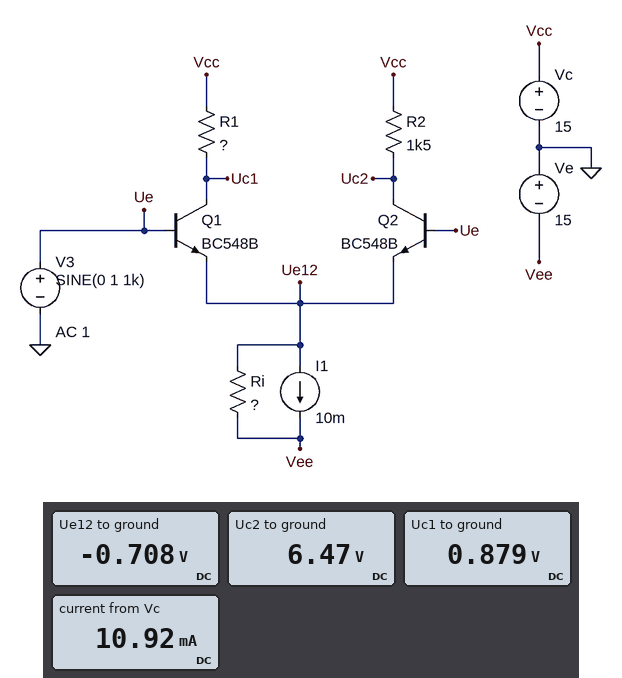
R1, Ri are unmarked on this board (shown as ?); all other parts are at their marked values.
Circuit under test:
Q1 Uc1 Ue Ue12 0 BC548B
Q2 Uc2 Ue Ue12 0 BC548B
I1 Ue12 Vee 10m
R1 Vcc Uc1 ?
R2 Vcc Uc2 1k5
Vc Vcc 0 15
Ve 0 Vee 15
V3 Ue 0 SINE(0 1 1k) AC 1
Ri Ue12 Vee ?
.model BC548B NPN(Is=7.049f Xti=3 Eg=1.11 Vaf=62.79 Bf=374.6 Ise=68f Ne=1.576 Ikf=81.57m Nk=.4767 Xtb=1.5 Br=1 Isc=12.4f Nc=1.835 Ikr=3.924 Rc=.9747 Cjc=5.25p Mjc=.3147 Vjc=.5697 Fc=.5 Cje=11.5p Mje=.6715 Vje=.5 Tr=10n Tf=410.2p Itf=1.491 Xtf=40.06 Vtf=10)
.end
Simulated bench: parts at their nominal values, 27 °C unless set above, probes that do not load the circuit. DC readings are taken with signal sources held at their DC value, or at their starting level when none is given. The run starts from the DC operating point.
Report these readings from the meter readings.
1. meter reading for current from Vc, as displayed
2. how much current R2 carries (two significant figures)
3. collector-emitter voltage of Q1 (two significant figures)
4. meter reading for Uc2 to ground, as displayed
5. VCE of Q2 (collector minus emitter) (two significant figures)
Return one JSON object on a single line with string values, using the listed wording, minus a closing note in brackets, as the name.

{"meter reading for current from Vc, as displayed": "10.92 mA", "how much current R2 carries": "5.7 mA", "collector-emitter voltage of Q1": "1.6 V", "meter reading for Uc2 to ground, as displayed": "6.47 V", "VCE of Q2 (collector minus emitter)": "7.2 V"}
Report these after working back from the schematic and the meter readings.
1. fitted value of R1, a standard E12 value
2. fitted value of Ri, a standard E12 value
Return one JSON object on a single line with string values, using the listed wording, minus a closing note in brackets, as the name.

{"fitted value of R1, a standard E12 value": "2.7 kΩ", "fitted value of Ri, a standard E12 value": "15 kΩ"}
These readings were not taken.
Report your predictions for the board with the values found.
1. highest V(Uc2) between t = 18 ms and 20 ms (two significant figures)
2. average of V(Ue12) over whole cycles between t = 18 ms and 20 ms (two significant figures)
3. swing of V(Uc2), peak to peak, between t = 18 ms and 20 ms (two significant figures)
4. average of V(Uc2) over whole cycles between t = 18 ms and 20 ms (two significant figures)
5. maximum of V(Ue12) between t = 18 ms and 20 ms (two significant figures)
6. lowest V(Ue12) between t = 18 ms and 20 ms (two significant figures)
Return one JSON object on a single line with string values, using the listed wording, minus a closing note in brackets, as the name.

{"highest V(Uc2) between t = 18 ms and 20 ms": "6.5 V", "average of V(Ue12) over whole cycles between t = 18 ms and 20 ms": "-710 mV", "swing of V(Uc2), peak to peak, between t = 18 ms and 20 ms": "120 mV", "average of V(Uc2) over whole cycles between t = 18 ms and 20 ms": "6.5 V", "maximum of V(Ue12) between t = 18 ms and 20 ms": "290 mV", "lowest V(Ue12) between t = 18 ms and 20 ms": "-1.7 V"}
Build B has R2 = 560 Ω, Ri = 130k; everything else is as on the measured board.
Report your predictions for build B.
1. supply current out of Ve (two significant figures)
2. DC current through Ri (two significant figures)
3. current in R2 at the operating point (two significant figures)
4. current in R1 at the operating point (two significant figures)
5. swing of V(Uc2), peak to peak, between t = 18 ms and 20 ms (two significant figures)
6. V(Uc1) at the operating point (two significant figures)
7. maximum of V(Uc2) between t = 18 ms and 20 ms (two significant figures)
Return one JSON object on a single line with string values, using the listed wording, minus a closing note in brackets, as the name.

{"supply current out of Ve": "10 mA", "DC current through Ri": "110 µA", "current in R2 at the operating point": "5.4 mA", "current in R1 at the operating point": "4.7 mA", "swing of V(Uc2), peak to peak, between t = 18 ms and 20 ms": "9.6 mV", "V(Uc1) at the operating point": "2.3 V", "maximum of V(Uc2) between t = 18 ms and 20 ms": "12 V"}
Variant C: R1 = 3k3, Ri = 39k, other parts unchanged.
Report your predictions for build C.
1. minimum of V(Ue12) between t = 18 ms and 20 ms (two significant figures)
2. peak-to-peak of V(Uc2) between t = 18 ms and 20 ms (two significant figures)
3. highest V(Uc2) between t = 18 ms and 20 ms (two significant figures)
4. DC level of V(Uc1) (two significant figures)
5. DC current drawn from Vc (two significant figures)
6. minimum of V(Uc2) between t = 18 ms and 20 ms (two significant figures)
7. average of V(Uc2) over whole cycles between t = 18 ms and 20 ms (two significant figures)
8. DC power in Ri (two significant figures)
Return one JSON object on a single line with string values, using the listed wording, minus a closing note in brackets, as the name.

{"minimum of V(Ue12) between t = 18 ms and 20 ms": "-1.7 V", "peak-to-peak of V(Uc2) between t = 18 ms and 20 ms": "200 mV", "highest V(Uc2) between t = 18 ms and 20 ms": "6.8 V", "DC level of V(Uc1)": "-600 mV", "DC current drawn from Vc": "10 mA", "minimum of V(Uc2) between t = 18 ms and 20 ms": "6.6 V", "average of V(Uc2) over whole cycles between t = 18 ms and 20 ms": "6.7 V", "DC power in Ri": "5.2 mW"}
